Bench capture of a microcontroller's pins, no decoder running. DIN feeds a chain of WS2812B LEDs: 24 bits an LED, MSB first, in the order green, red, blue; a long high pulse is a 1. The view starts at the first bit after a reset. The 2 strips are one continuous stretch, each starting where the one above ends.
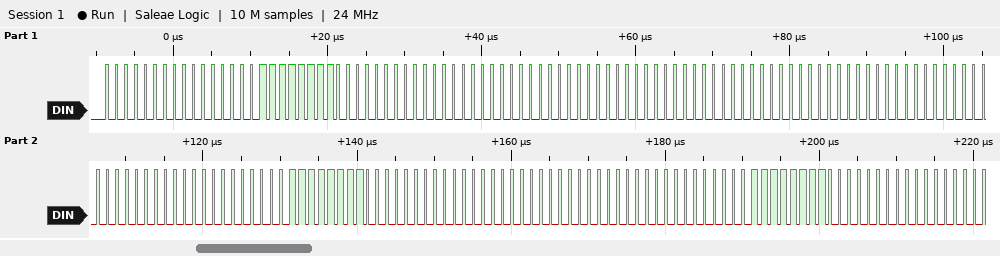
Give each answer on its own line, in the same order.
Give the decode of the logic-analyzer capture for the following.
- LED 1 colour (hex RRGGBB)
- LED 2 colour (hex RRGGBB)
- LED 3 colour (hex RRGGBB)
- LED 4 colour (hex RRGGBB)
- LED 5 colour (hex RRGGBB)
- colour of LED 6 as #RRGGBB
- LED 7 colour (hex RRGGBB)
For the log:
#0000FF
#000000
#000000
#000000
#0000FF
#000000
#0000FF
